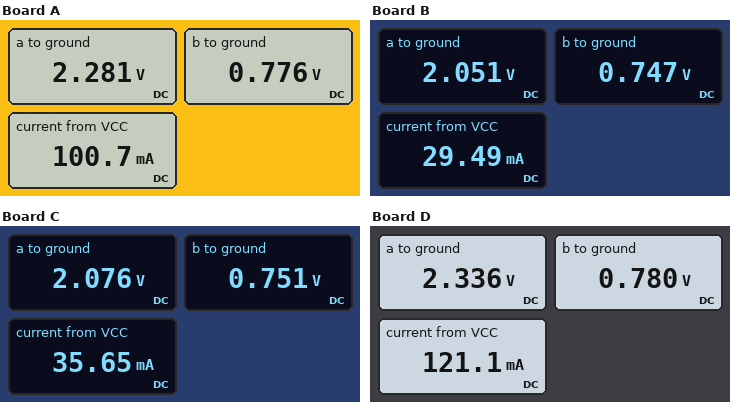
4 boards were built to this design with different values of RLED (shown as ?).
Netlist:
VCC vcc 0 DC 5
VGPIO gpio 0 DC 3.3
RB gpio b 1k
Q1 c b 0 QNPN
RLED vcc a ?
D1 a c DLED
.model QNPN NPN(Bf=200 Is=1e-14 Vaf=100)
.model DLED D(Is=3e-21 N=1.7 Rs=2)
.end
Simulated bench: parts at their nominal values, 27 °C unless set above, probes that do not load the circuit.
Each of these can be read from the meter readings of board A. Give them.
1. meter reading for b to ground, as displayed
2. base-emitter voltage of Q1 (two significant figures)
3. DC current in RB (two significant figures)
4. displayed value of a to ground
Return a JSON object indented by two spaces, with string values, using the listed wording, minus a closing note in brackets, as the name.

{
  "meter reading for b to ground, as displayed": "0.776 V",
  "base-emitter voltage of Q1": "780 mV",
  "DC current in RB": "2.5 mA",
  "displayed value of a to ground": "2.281 V"
}
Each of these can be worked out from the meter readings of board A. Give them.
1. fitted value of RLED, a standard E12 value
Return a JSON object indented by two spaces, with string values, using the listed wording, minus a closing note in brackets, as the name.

{
  "fitted value of RLED, a standard E12 value": "27 Ω"
}
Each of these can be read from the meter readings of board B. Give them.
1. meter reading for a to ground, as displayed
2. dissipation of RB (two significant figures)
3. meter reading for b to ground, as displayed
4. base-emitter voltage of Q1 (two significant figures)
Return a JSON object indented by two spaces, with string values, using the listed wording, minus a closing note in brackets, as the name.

{
  "meter reading for a to ground, as displayed": "2.051 V",
  "dissipation of RB": "6.5 mW",
  "meter reading for b to ground, as displayed": "0.747 V",
  "base-emitter voltage of Q1": "750 mV"
}
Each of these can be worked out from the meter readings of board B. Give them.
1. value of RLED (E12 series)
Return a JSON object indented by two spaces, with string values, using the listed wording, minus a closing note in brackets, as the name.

{
  "value of RLED": "100 Ω"
}
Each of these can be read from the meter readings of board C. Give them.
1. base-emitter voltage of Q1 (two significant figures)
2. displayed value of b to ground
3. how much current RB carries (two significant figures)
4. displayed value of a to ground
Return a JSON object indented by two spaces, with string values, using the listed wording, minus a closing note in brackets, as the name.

{
  "base-emitter voltage of Q1": "750 mV",
  "displayed value of b to ground": "0.751 V",
  "how much current RB carries": "2.5 mA",
  "displayed value of a to ground": "2.076 V"
}
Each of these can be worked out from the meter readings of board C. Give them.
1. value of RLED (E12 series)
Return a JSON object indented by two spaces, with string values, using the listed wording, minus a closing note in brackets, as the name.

{
  "value of RLED": "82 Ω"
}
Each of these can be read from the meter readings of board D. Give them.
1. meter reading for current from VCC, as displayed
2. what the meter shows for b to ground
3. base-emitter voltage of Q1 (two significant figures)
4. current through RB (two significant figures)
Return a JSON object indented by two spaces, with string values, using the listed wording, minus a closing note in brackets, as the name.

{
  "meter reading for current from VCC, as displayed": "121.1 mA",
  "what the meter shows for b to ground": "0.780 V",
  "base-emitter voltage of Q1": "780 mV",
  "current through RB": "2.5 mA"
}
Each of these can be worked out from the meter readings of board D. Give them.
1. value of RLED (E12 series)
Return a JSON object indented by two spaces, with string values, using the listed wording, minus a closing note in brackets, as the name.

{
  "value of RLED": "22 Ω"
}
